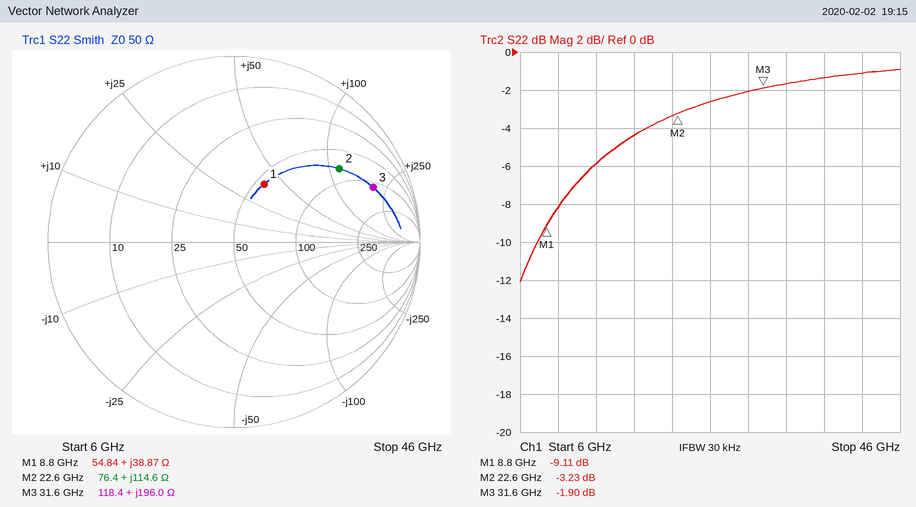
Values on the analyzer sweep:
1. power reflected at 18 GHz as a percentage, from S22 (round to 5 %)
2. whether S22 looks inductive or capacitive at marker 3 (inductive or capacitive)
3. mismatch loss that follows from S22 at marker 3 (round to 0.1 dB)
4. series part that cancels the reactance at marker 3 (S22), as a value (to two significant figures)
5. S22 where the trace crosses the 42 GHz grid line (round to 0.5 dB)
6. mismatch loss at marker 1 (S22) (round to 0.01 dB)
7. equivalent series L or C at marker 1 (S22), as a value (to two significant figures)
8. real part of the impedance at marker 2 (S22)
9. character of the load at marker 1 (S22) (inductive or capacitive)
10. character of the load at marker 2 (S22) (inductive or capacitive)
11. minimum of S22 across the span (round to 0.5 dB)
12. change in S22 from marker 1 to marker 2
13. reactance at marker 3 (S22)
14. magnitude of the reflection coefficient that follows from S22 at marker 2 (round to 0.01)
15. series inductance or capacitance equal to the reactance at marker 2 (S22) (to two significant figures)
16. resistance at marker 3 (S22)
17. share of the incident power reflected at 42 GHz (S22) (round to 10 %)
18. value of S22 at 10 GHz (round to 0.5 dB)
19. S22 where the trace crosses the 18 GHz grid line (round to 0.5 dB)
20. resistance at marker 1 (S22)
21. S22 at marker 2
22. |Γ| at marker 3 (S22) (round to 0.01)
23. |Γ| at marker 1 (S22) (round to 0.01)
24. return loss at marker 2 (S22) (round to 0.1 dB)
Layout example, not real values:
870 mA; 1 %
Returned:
35 %; inductive; 4.5 dB; 26 fF; -1.0 dB; 0.57 dB; 700 pH; 76.4 Ω; inductive; inductive; -12.0 dB; 5.88 dB; +196.0 Ω; 0.69; 810 pH; 118.4 Ω; 80 %; -8.0 dB; -4.5 dB; 54.84 Ω; -3.23 dB; 0.80; 0.35; 3.2 dB
